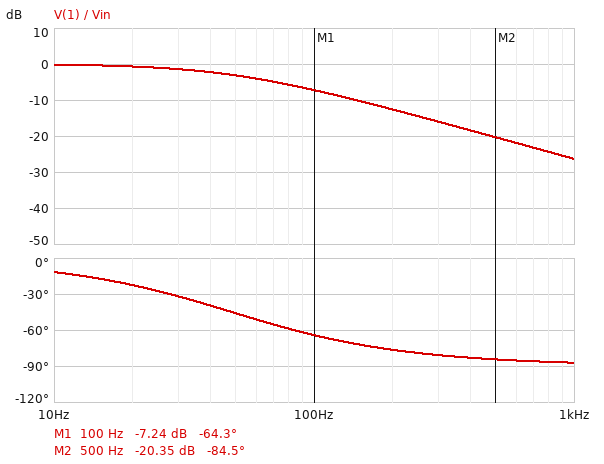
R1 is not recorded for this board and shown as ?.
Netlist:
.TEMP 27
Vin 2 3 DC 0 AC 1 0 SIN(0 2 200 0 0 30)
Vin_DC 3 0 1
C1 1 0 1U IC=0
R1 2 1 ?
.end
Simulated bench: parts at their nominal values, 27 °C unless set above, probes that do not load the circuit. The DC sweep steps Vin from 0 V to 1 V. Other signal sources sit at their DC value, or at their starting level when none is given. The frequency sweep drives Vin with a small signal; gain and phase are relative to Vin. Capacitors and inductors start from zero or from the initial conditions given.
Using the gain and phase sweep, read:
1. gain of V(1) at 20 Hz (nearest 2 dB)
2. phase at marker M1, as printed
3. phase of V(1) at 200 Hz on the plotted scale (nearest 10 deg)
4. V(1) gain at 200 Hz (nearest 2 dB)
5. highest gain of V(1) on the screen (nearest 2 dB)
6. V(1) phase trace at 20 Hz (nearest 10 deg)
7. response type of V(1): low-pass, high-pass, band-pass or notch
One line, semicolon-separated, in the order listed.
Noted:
0 dB; -64.3 deg; -80 deg; -12 dB; 0 dB; -20 deg; low-pass
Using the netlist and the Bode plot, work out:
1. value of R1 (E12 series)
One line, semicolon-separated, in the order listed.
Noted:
3.3 kΩ
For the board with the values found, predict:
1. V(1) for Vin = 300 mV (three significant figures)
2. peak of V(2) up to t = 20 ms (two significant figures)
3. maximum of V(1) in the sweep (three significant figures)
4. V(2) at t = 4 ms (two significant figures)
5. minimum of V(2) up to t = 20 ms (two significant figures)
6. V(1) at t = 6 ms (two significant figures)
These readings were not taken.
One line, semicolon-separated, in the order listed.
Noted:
1.30 V; 3.0 V; 2.00 V; -340 mV; -1.0 V; 1.1 V
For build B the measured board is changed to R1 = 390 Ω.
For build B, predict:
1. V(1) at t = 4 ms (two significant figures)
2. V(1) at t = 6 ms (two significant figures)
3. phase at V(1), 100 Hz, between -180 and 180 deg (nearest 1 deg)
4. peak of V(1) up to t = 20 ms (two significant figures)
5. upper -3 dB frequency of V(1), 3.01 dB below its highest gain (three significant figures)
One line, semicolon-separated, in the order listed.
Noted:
-670 mV; 2.7 V; -14 deg; 2.8 V; 408 Hz
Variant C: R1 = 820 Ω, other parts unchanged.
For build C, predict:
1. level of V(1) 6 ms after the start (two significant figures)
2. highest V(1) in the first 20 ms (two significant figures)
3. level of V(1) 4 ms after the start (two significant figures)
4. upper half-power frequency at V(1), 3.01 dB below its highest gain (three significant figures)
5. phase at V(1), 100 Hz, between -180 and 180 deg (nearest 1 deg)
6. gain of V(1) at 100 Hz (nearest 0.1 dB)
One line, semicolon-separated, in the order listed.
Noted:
2.2 V; 2.4 V; -400 mV; 194 Hz; -27 deg; -1.0 dB
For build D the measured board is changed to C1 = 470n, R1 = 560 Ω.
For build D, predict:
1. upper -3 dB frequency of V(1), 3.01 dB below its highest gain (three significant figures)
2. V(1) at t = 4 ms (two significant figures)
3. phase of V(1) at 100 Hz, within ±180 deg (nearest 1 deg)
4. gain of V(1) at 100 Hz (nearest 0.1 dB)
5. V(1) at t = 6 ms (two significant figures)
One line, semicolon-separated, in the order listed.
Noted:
605 Hz; -650 mV; -9 deg; -0.1 dB; 2.9 V
